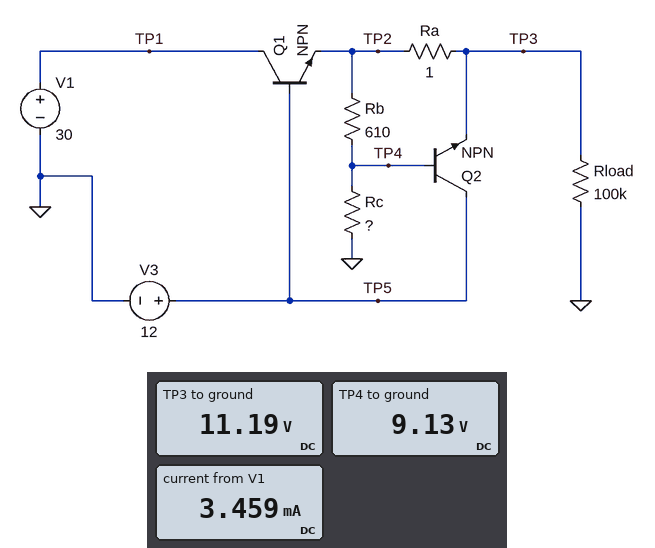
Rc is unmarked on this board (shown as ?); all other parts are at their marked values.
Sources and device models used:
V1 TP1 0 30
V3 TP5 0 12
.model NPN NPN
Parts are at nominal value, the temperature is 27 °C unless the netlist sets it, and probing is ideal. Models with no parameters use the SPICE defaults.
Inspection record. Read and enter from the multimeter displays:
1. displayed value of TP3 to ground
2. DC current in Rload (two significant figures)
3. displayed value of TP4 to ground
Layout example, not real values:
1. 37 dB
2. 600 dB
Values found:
1. 11.19 V
2. 110 µA
3. 9.13 V
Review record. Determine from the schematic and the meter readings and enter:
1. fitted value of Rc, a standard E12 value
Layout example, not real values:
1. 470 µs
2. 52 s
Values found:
1. 2.7 kΩ
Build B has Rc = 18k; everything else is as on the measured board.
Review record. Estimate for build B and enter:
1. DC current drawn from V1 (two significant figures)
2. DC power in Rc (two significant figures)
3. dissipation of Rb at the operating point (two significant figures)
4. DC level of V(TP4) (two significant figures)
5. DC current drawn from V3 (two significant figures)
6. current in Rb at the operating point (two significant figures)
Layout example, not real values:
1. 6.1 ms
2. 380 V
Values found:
1. 710 µA
2. 6.6 mW
3. 220 µW
4. 11 V
5. 7.1 µA
6. 600 µA
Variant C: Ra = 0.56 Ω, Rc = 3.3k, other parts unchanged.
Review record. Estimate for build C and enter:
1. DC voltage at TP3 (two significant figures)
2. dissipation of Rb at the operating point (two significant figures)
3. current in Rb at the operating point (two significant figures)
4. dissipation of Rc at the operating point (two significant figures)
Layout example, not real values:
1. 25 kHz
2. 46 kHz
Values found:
1. 11 V
2. 5.0 mW
3. 2.9 mA
4. 27 mW
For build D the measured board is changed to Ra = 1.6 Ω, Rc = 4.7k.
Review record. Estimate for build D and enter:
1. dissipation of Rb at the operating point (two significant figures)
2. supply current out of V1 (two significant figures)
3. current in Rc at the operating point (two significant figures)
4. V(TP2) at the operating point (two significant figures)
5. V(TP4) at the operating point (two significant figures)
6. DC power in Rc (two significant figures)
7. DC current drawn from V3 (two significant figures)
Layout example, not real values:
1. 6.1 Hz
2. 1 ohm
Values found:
1. 2.7 mW
2. 2.2 mA
3. 2.1 mA
4. 11 V
5. 9.9 V
6. 21 mW
7. 22 µA
